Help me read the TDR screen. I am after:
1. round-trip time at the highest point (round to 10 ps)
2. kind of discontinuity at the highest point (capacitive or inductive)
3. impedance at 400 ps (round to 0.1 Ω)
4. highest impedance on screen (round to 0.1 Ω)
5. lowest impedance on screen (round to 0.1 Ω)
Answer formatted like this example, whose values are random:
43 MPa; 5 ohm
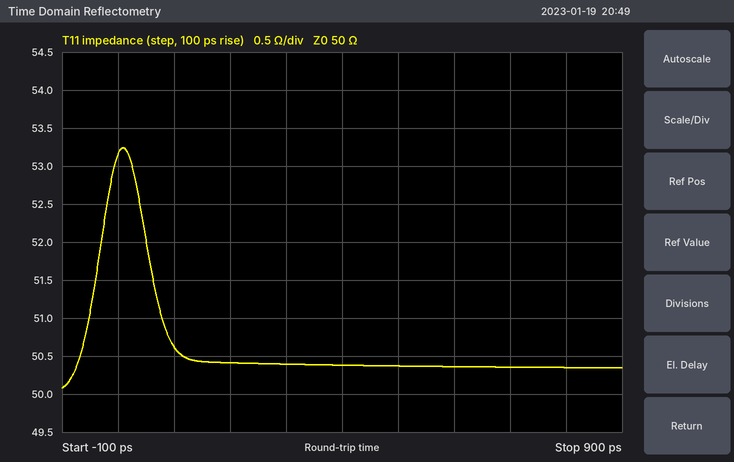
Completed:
10 ps; inductive; 50.4 Ω; 53.2 Ω; 50.1 Ω
